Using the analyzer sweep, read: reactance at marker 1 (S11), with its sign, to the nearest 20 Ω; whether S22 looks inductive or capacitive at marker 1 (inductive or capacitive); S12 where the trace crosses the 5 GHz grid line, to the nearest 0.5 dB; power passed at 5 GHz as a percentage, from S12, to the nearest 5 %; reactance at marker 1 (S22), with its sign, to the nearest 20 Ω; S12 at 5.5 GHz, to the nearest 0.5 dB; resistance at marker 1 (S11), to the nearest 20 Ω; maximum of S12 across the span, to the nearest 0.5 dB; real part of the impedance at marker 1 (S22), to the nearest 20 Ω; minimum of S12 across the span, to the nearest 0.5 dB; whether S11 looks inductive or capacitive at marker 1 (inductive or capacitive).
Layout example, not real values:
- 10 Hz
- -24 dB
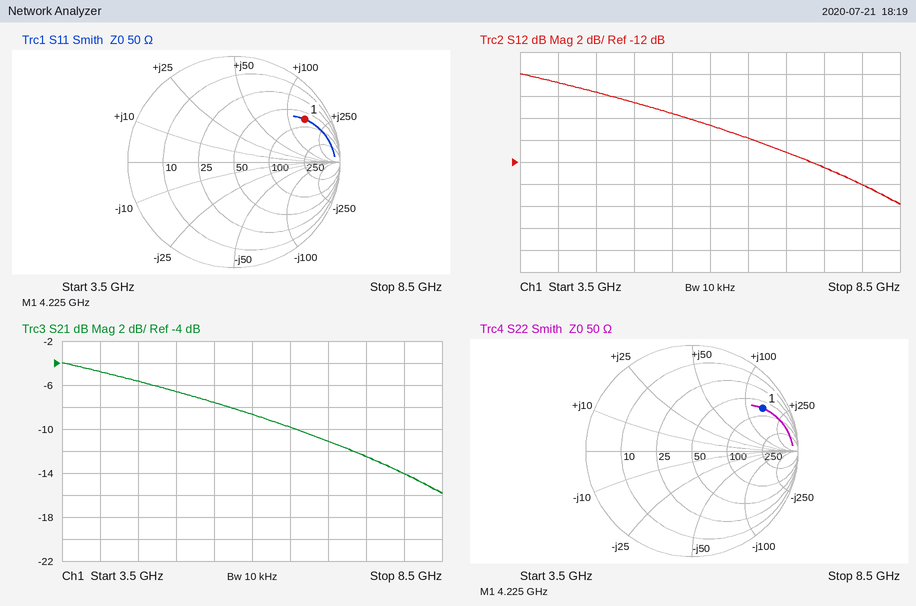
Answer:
- +140 Ω
- inductive
- -6.5 dB
- 20 %
- +140 Ω
- -7.5 dB
- 80 Ω
- -4.0 dB
- 80 Ω
- -16.0 dB
- inductive
